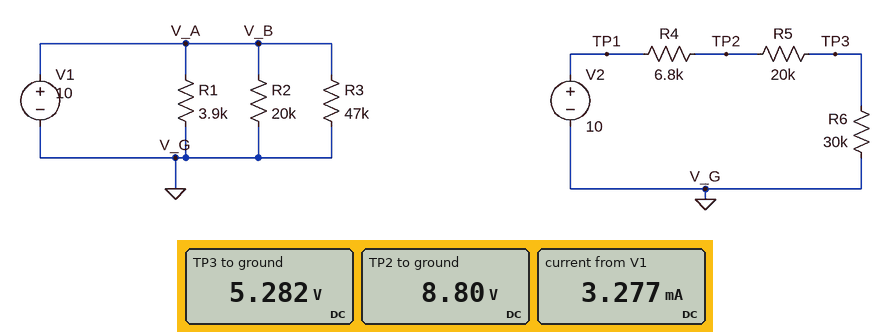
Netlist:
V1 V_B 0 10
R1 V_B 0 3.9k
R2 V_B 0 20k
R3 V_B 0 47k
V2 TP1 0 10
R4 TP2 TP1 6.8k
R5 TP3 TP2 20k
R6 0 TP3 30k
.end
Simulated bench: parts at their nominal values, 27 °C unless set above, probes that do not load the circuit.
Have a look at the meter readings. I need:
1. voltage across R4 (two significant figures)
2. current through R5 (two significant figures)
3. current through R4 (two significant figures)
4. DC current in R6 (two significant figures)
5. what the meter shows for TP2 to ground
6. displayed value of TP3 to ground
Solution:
1.2 V
180 µA
180 µA
180 µA
8.80 V
5.282 V
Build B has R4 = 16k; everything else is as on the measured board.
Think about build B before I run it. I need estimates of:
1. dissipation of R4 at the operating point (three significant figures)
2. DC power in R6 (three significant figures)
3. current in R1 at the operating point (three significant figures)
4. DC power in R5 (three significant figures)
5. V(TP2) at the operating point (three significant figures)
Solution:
367 µW
689 µW
2.56 mA
459 µW
7.58 V
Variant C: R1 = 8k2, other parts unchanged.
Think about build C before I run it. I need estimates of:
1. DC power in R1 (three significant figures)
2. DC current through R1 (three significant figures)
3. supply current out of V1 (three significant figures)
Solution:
12.2 mW
1.22 mA
1.93 mA
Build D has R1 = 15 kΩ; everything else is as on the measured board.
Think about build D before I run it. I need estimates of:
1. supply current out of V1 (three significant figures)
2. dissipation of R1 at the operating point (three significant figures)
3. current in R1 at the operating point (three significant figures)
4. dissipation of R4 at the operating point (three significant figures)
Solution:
1.38 mA
6.67 mW
667 µA
211 µW
